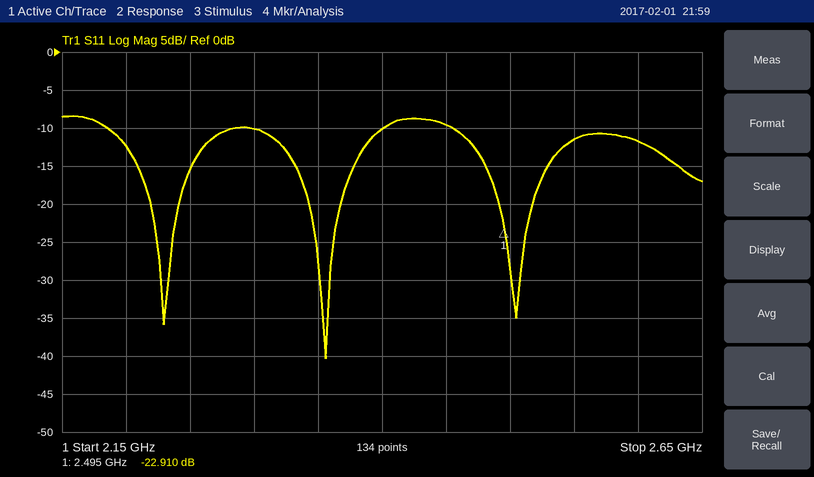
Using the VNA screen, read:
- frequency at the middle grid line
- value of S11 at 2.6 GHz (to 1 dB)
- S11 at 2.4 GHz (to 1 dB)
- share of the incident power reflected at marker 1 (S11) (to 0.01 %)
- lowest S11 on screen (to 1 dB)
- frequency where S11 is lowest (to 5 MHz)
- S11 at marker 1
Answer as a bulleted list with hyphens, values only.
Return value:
- 2.4 GHz
- -12 dB
- -10 dB
- 0.51 %
- -40 dB
- 2.355 GHz
- -22.910 dB
